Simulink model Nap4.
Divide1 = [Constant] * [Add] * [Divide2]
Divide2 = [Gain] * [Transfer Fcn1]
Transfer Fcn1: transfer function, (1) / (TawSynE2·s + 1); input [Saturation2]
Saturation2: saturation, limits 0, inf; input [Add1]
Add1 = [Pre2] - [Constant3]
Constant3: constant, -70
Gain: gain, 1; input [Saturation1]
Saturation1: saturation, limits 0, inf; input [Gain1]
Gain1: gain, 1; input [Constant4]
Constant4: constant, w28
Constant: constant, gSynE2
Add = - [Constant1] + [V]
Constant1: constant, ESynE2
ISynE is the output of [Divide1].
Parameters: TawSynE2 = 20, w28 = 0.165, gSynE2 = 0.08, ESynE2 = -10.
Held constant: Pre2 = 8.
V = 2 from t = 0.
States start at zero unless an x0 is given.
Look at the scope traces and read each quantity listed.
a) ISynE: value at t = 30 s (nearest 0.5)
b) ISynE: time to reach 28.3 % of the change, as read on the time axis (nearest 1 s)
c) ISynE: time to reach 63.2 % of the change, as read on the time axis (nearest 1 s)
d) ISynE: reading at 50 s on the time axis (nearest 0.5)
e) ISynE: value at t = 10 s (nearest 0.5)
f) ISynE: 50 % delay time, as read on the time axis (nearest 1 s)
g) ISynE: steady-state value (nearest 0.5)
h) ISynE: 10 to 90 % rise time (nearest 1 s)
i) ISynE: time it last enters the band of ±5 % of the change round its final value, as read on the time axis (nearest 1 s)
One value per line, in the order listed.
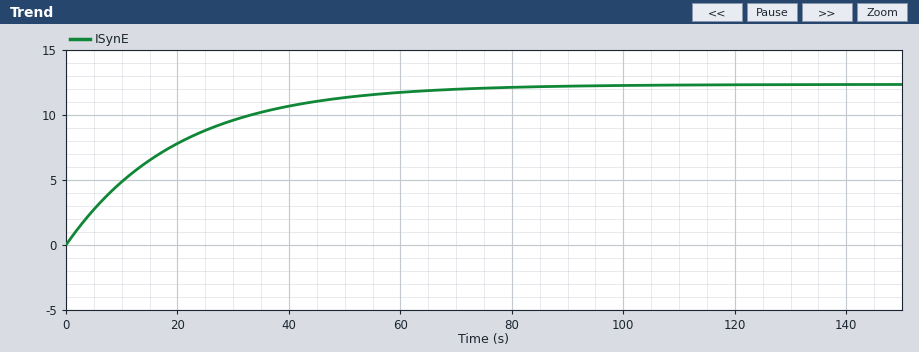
9.5
7 s
20 s
11.5
5.0
14 s
12.5
44 s
60 s
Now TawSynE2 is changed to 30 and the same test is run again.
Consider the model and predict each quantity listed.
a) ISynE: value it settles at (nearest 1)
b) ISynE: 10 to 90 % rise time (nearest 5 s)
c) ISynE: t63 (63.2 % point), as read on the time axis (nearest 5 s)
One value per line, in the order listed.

12
65 s
30 s
